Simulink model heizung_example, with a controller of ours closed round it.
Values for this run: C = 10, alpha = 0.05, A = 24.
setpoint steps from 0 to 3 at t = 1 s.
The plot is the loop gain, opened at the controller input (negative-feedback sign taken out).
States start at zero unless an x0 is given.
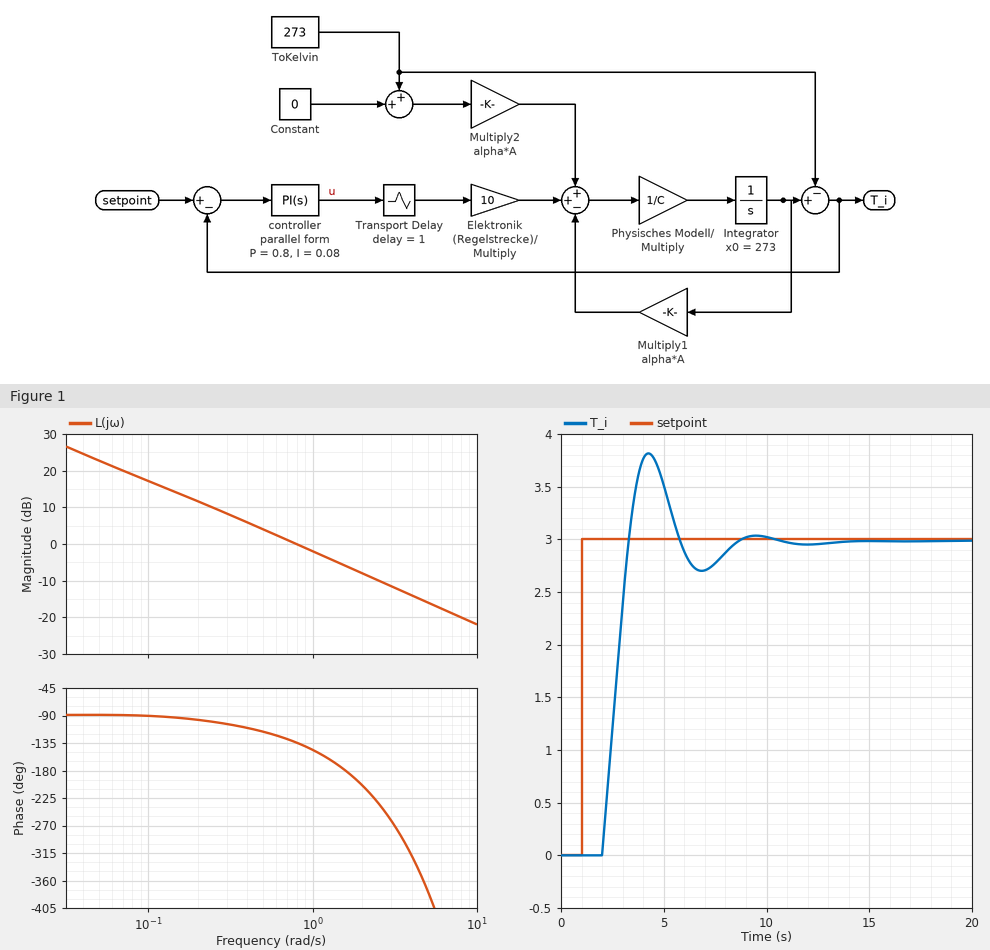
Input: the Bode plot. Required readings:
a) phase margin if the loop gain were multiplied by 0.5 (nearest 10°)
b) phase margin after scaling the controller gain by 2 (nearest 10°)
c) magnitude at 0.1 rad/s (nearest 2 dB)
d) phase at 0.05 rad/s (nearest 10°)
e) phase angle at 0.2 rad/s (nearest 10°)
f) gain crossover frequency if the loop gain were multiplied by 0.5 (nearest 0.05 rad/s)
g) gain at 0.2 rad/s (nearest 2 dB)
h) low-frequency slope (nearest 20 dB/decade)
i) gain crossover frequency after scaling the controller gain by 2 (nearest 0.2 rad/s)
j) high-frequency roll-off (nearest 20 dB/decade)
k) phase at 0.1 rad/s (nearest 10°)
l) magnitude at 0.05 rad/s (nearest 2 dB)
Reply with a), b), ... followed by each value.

a) 70°
b) 0°
c) 18 dB
d) -90°
e) -100°
f) 0.40 rad/s
g) 12 dB
h) -20 dB/decade
i) 1.6 rad/s
j) -20 dB/decade
k) -90°
l) 22 dB
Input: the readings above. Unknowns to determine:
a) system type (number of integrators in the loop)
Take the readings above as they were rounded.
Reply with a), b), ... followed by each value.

a) 1
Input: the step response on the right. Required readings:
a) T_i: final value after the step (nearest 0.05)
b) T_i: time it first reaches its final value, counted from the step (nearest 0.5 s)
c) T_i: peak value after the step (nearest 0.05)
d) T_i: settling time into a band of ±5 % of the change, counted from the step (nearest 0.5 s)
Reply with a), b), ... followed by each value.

a) 3.00
b) 2.5 s
c) 3.80
d) 7.0 s
